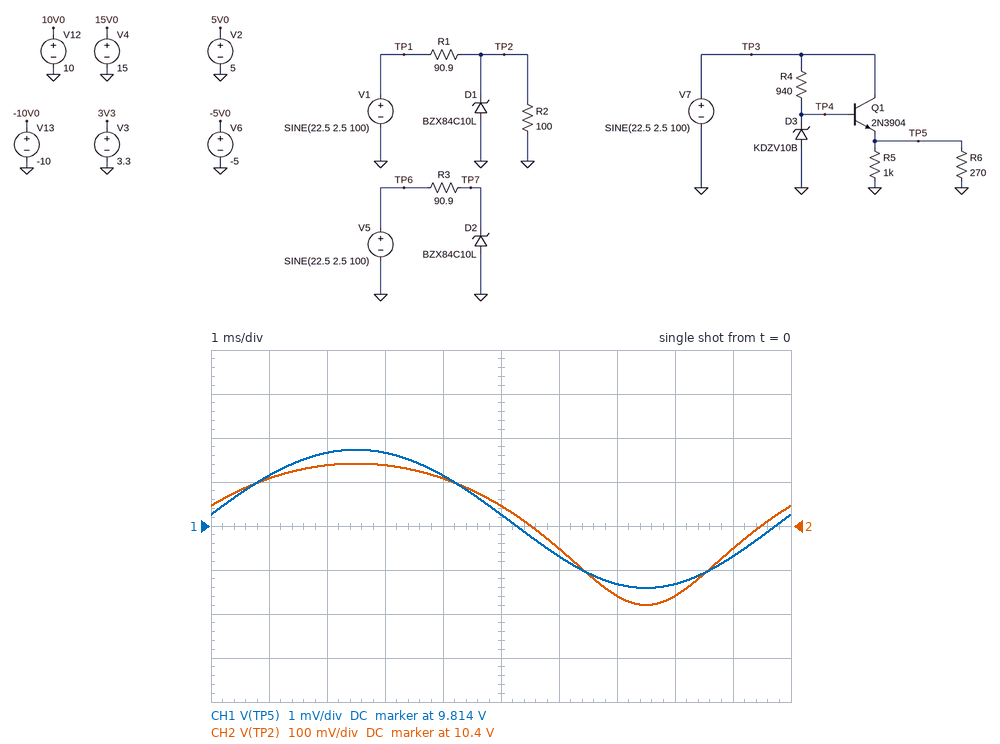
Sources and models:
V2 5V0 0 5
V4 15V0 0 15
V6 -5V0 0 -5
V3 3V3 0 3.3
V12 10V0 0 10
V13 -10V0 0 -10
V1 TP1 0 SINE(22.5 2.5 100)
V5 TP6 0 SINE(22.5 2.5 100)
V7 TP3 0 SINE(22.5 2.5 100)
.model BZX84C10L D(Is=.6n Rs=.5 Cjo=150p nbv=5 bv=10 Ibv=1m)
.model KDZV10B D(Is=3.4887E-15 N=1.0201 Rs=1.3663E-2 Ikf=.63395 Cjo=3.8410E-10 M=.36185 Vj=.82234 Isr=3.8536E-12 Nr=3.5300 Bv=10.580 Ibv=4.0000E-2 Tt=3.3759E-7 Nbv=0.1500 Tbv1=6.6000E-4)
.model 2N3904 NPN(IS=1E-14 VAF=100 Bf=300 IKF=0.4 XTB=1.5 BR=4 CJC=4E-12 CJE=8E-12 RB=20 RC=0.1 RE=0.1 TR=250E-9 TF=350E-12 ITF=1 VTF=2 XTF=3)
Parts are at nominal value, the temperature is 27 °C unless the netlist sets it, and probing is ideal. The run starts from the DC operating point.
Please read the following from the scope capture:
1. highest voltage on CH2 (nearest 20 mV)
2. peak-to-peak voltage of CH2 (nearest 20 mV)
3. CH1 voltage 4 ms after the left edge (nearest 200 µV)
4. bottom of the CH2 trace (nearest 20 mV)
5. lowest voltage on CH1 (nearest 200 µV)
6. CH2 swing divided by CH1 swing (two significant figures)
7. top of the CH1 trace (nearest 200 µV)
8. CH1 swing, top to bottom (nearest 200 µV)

10.54 V
320 mV
9.8152 V
10.22 V
9.8126 V
100
9.8158 V
3.2 mV
